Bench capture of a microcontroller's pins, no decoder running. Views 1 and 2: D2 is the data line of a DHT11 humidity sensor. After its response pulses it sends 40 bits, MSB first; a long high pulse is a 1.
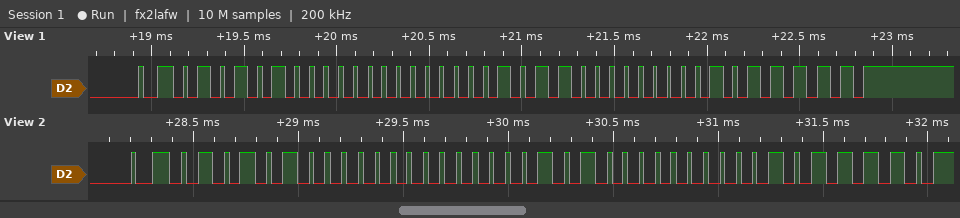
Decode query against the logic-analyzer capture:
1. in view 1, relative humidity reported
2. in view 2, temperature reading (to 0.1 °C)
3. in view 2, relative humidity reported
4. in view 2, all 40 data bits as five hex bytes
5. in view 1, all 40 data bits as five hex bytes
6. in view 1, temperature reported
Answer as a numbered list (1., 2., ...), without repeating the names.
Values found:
1. 84 %
2. 10.0 °C
3. 84 %
4. 54 00 0A 00 5E
5. 54 00 0B 00 5F
6. 11.0 °C
